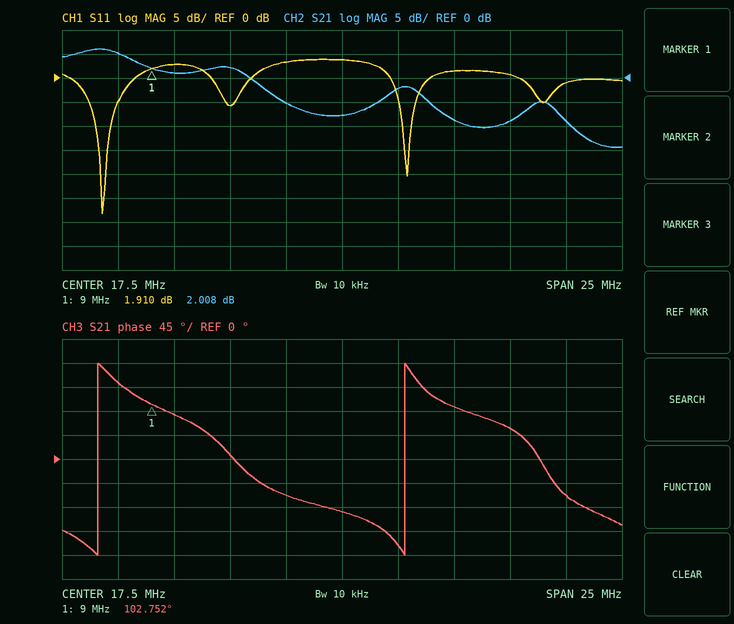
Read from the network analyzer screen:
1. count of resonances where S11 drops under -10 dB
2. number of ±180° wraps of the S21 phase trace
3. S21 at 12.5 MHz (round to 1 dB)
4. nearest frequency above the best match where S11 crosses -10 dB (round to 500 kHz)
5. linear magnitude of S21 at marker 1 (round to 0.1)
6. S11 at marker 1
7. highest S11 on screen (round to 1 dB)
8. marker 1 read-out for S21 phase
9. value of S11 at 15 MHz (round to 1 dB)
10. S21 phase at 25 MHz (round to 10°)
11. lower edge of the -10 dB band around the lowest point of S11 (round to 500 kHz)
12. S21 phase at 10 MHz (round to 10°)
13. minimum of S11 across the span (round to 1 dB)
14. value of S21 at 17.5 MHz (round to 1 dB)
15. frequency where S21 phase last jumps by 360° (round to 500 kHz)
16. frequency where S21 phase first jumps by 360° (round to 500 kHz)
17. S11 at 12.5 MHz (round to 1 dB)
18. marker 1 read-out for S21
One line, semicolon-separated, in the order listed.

2; 2; 2 dB; 7.0 MHz; 1.3; 1.910 dB; 4 dB; 102.752°; 3 dB; 60°; 6.5 MHz; 80°; -28 dB; -8 dB; 20.5 MHz; 6.5 MHz; -6 dB; 2.008 dB
